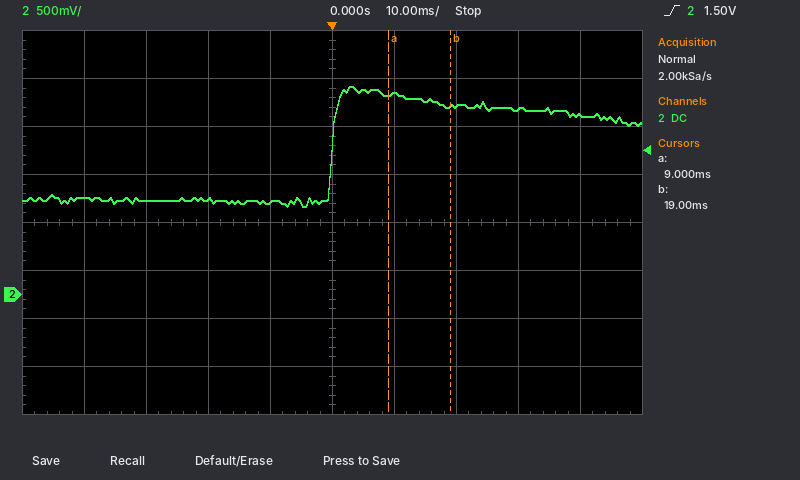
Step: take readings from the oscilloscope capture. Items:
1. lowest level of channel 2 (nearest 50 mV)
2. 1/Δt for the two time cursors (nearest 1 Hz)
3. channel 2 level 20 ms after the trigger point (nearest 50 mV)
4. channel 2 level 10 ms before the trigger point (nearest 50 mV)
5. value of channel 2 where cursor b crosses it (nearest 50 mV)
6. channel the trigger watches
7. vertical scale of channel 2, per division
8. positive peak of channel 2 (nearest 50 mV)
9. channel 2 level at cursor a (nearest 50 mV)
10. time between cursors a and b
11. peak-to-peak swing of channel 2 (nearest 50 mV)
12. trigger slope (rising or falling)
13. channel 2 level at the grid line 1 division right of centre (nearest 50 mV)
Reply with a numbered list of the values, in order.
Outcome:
1. 900 mV
2. 100 Hz
3. 1.95 V
4. 950 mV
5. 1.95 V
6. channel 2
7. 500 mV
8. 2.15 V
9. 2.10 V
10. 10 ms
11. 1.25 V
12. rising
13. 2.10 V
